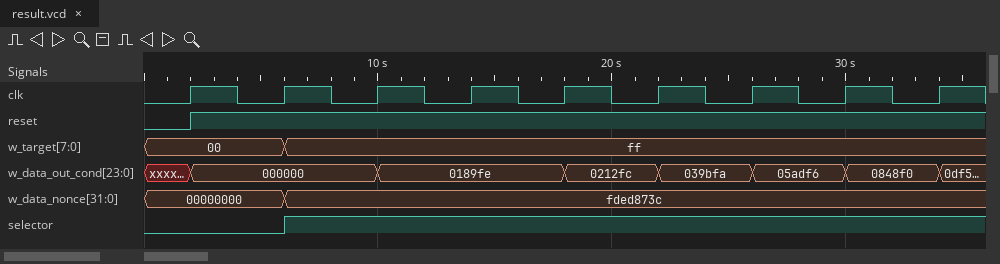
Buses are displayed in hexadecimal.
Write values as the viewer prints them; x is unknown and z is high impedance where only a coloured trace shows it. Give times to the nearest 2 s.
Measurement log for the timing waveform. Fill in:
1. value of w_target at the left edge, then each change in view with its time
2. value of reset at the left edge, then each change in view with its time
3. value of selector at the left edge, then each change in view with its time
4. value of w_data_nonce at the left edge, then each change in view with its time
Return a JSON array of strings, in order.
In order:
["00, ff at 6 s", "0, 1 at 2 s", "0, 1 at 6 s", "00000000, fded873c at 6 s"]
